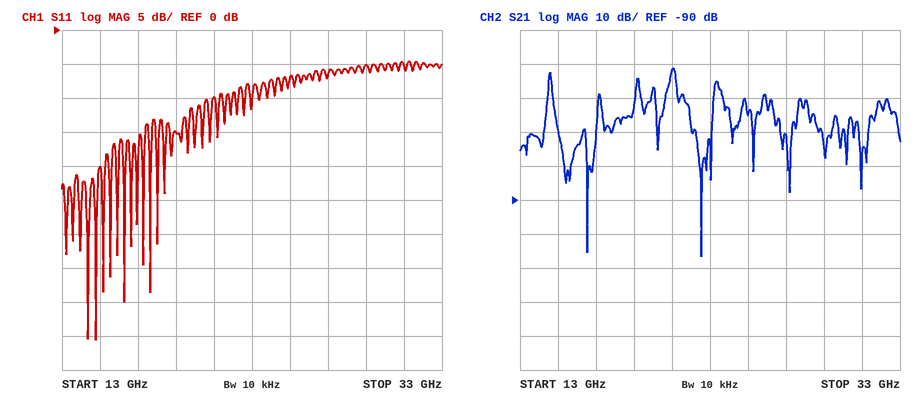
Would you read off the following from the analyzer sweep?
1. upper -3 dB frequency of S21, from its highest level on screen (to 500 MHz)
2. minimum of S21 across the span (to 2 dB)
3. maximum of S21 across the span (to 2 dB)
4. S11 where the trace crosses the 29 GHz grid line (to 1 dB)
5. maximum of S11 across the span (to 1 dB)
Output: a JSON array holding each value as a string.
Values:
["21.0 GHz", "-106 dB", "-52 dB", "-5 dB", "-5 dB"]
